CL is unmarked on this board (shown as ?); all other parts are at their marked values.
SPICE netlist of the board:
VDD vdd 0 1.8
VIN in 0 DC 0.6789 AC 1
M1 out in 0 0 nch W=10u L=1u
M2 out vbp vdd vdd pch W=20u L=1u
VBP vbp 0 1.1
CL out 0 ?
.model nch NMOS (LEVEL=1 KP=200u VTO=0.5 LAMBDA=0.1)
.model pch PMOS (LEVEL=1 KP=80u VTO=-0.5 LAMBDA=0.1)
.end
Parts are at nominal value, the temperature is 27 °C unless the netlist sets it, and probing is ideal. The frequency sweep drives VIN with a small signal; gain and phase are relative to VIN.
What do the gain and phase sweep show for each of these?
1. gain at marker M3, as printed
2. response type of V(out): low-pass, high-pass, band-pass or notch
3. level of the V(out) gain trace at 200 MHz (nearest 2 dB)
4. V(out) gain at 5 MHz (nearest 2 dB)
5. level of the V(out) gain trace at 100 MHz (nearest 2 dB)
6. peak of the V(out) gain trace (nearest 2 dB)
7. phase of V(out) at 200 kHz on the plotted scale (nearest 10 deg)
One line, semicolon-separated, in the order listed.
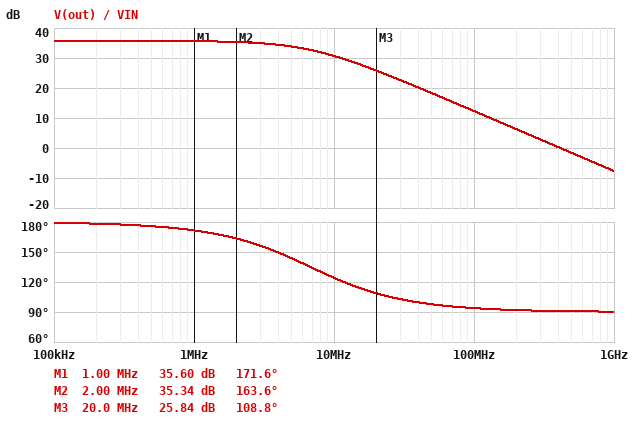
25.84 dB; low-pass; 6 dB; 34 dB; 12 dB; 36 dB; 180 deg
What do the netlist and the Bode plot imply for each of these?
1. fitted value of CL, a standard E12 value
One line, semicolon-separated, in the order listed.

150 fF
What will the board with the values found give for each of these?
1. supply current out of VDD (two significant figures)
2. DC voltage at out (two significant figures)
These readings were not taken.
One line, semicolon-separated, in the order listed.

35 µA; 900 mV
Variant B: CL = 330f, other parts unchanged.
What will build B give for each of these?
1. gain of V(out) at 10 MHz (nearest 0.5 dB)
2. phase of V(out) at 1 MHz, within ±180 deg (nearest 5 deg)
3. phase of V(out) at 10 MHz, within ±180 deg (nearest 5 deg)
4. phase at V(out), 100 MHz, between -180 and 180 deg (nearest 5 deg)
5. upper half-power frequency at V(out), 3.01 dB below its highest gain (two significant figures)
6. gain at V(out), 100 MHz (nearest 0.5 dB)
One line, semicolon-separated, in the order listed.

25.0 dB; 160 deg; 105 deg; 90 deg; 3.1 MHz; 5.5 dB
